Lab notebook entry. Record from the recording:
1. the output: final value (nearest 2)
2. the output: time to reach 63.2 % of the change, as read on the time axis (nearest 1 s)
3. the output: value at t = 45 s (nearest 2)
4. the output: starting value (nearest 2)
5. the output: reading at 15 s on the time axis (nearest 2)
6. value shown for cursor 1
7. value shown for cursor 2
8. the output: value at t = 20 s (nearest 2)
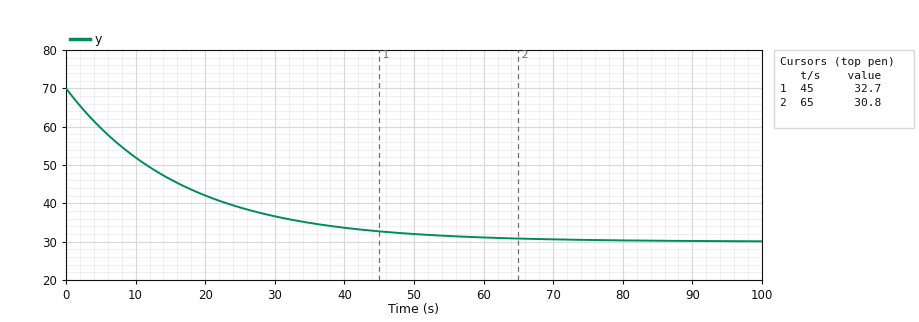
30
17 s
32
70
46
32.7
30.8
42
